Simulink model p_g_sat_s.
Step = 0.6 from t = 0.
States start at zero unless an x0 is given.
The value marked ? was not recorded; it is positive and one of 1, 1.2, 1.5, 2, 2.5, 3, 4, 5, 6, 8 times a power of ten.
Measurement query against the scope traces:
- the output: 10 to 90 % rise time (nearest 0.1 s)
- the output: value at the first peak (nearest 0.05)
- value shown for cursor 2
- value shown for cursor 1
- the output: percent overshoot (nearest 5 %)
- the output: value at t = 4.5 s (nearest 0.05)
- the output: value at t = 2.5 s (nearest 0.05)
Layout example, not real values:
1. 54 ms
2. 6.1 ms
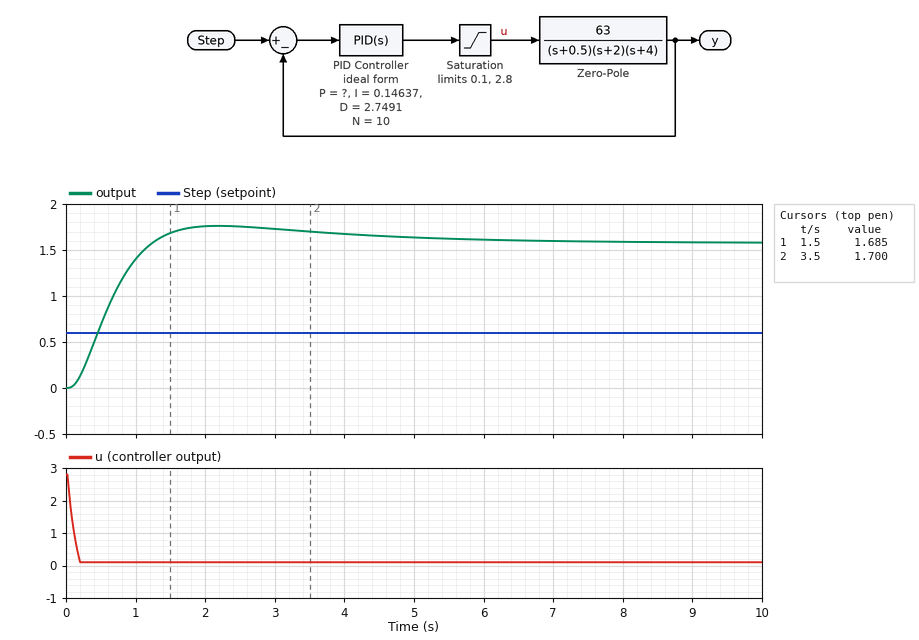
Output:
1. 0.8 s
2. 1.75
3. 1.700
4. 1.685
5. 10 %
6. 1.65
7. 1.75
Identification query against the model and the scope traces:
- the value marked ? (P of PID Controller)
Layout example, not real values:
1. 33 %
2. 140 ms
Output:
1. 0.2
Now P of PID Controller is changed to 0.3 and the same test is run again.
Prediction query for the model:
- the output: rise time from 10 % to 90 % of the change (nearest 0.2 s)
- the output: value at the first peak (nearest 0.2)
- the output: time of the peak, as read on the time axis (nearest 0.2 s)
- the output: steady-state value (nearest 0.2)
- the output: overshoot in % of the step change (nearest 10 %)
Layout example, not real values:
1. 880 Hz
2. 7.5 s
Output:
1. 0.6 s
2. 2.0
3. 1.8 s
4. 1.6
5. 30 %
